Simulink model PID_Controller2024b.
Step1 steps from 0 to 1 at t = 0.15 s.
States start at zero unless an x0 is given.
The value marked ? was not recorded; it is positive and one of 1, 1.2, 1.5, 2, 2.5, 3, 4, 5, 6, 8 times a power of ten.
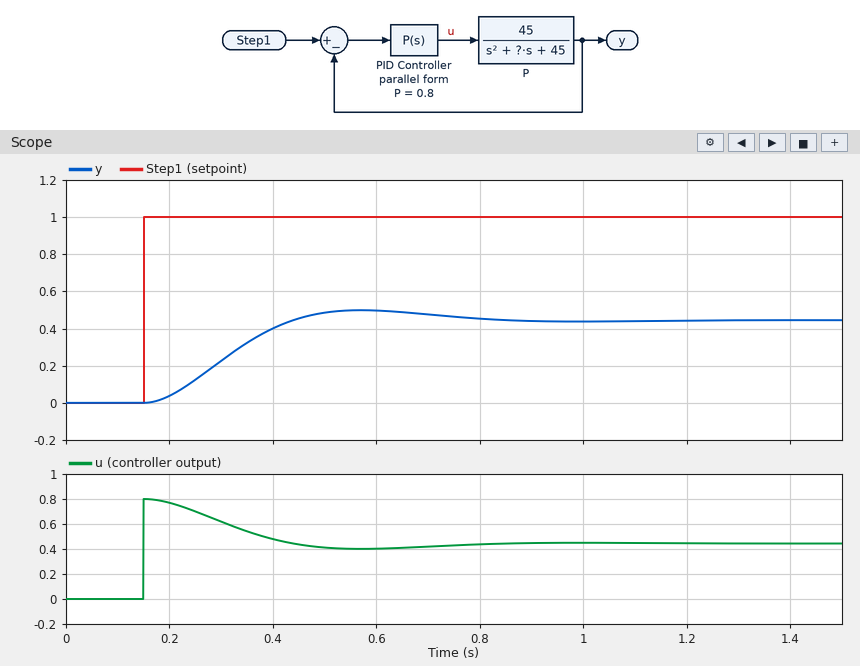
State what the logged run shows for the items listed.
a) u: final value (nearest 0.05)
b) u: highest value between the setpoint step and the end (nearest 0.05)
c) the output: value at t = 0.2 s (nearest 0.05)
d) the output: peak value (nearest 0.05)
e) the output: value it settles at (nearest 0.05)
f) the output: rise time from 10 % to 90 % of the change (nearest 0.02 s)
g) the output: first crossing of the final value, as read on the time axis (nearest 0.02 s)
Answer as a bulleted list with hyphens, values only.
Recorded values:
- 0.45
- 0.80
- 0.05
- 0.50
- 0.45
- 0.20 s
- 0.44 s
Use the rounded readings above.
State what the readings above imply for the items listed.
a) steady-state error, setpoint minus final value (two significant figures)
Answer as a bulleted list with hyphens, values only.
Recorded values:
- 0.55
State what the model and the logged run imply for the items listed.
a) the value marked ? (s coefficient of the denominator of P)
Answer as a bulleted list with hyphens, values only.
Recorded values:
- 10
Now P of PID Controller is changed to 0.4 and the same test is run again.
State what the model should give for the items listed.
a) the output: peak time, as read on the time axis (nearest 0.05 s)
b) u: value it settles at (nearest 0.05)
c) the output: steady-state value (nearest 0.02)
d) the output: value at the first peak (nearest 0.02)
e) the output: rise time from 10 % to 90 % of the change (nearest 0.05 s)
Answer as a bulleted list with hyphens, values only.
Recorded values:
- 0.65 s
- 0.30
- 0.28
- 0.30
- 0.25 s
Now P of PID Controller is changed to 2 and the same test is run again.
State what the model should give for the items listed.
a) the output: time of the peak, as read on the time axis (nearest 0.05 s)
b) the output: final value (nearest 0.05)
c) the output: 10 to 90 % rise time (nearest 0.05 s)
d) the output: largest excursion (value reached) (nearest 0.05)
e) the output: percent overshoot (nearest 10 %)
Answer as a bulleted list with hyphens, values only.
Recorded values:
- 0.45 s
- 0.65
- 0.15 s
- 0.80
- 20 %
